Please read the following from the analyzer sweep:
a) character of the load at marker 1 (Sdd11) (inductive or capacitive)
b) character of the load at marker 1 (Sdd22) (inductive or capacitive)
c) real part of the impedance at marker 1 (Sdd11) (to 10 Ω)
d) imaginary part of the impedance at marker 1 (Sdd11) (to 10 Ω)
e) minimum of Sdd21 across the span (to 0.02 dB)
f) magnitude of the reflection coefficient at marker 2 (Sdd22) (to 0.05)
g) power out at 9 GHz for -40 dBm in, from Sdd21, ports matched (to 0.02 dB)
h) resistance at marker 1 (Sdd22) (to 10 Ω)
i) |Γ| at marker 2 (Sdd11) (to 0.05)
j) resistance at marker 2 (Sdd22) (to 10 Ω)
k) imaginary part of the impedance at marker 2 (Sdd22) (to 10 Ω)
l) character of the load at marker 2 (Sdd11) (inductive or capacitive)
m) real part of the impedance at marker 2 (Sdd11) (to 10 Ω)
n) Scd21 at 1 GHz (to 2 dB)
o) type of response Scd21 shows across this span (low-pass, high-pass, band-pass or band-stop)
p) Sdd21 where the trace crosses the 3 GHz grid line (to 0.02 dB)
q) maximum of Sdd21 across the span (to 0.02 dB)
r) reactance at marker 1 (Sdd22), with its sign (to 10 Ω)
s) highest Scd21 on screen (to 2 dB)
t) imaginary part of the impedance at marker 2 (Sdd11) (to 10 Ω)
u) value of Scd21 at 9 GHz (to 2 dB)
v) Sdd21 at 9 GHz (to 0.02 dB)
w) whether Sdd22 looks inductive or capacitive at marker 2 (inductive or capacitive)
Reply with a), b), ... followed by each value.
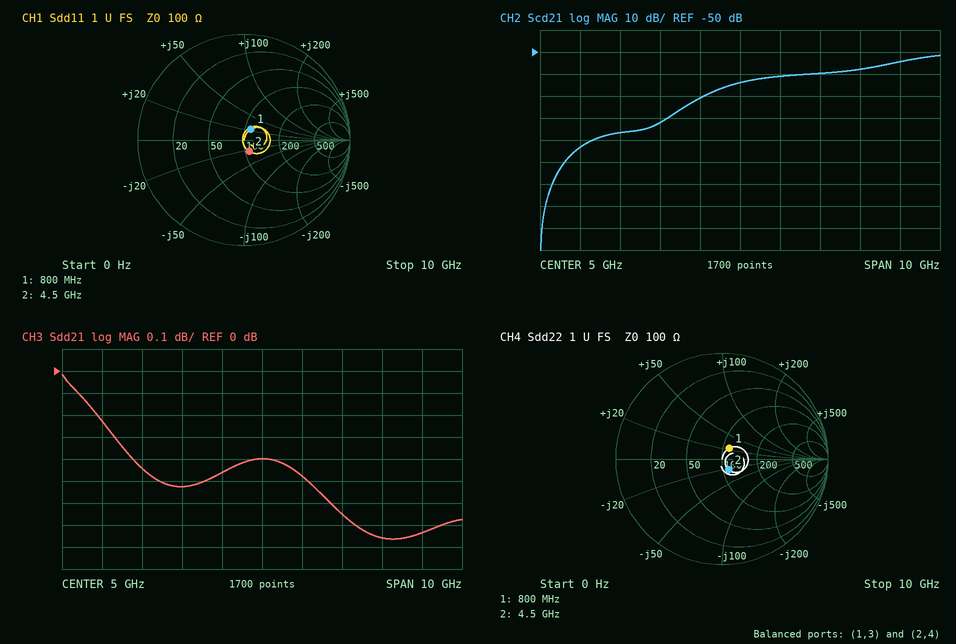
a) inductive
b) inductive
c) 110 Ω
d) +20 Ω
e) -0.76 dB
f) 0.10
g) -40.74 dBm
h) 110 Ω
i) 0.10
j) 110 Ω
k) -20 Ω
l) capacitive
m) 110 Ω
n) -94 dB
o) high-pass
p) -0.52 dB
q) -0.02 dB
r) +20 Ω
s) -52 dB
t) -20 Ω
u) -54 dB
v) -0.74 dB
w) capacitive
